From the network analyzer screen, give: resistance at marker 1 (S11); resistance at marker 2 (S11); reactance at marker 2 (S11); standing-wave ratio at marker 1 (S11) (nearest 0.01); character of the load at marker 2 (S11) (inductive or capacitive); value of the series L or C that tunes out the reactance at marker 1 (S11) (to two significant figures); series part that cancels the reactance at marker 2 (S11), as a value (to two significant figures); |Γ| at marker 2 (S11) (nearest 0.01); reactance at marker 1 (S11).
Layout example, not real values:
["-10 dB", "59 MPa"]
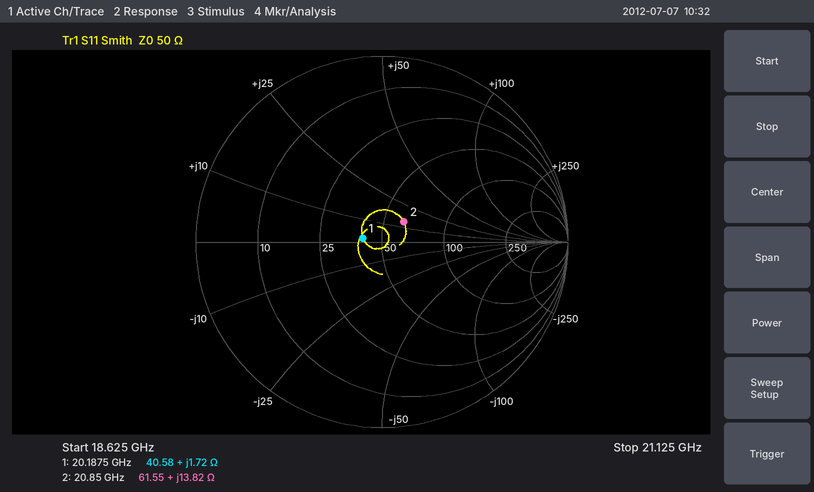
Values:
["40.58 Ω", "61.55 Ω", "+13.82 Ω", "1.24", "inductive", "4.6 pF", "550 fF", "0.16", "+1.72 Ω"]
